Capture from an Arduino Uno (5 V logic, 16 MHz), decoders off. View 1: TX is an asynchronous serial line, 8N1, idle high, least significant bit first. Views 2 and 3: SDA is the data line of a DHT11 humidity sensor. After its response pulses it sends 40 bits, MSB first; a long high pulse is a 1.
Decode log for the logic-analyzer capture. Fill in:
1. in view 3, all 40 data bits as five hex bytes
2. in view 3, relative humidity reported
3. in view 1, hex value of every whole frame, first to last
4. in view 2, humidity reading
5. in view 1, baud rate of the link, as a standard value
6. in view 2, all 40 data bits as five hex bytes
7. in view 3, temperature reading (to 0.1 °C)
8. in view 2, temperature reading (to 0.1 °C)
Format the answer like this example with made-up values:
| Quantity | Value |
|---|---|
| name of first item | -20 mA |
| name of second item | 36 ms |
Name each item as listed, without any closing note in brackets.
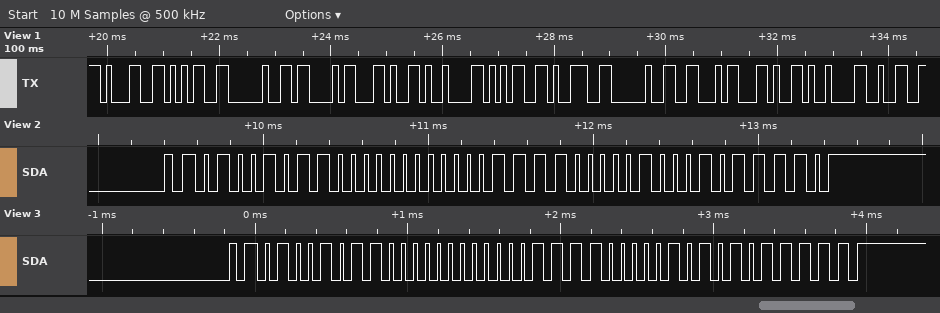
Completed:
| Quantity | Value |
|---|---|
| in view 3, all 40 data bits as five hex bytes | 4B 00 0F 05 5F |
| in view 3, relative humidity reported | 75 % |
| in view 1, hex value of every whole frame, first to last | 31 35 20 43 2C 09 35 39 20 46 2C 09 32 |
| in view 2, humidity reading | 75 % |
| in view 1, baud rate of the link, as a standard value | 9600 baud |
| in view 2, all 40 data bits as five hex bytes | 4B 00 0F 04 5E |
| in view 3, temperature reading | 15.5 °C |
| in view 2, temperature reading | 15.4 °C |
